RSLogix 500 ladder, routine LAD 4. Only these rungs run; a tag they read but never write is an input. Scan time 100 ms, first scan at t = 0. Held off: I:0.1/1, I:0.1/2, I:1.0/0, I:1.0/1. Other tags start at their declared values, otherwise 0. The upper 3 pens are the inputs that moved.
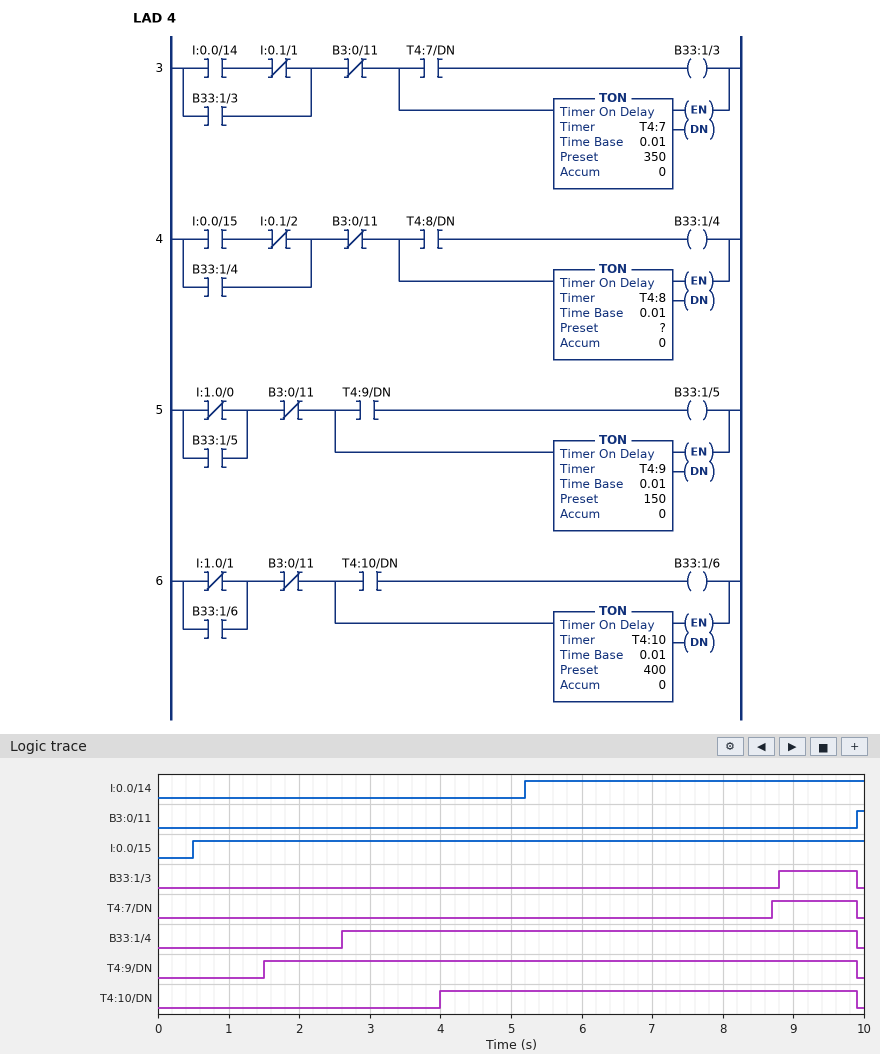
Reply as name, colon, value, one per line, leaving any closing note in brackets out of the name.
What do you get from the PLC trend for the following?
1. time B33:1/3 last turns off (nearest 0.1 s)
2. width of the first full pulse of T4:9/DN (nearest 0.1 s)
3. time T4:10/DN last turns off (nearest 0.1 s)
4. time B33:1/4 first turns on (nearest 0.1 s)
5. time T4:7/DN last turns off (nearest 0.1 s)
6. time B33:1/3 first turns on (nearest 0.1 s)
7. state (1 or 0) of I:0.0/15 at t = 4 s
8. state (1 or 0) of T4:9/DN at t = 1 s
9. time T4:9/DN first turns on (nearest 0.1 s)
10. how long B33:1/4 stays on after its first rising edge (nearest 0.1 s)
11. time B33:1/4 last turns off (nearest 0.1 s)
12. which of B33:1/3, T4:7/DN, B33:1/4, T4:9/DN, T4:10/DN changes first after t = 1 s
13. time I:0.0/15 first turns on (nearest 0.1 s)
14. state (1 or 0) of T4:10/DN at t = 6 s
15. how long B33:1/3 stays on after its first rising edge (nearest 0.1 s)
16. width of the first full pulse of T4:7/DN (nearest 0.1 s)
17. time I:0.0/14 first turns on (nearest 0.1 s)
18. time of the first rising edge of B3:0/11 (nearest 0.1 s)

time B33:1/3 last turns off: 9.9 s
width of the first full pulse of T4:9/DN: 8.4 s
time T4:10/DN last turns off: 9.9 s
time B33:1/4 first turns on: 2.6 s
time T4:7/DN last turns off: 9.9 s
time B33:1/3 first turns on: 8.8 s
state (1 or 0) of I:0.0/15 at t = 4 s: 1
state (1 or 0) of T4:9/DN at t = 1 s: 0
time T4:9/DN first turns on: 1.5 s
how long B33:1/4 stays on after its first rising edge: 7.3 s
time B33:1/4 last turns off: 9.9 s
which of B33:1/3, T4:7/DN, B33:1/4, T4:9/DN, T4:10/DN changes first after t = 1 s: T4:9/DN
time I:0.0/15 first turns on: 0.5 s
state (1 or 0) of T4:10/DN at t = 6 s: 1
how long B33:1/3 stays on after its first rising edge: 1.1 s
width of the first full pulse of T4:7/DN: 1.2 s
time I:0.0/14 first turns on: 5.2 s
time of the first rising edge of B3:0/11: 9.9 s
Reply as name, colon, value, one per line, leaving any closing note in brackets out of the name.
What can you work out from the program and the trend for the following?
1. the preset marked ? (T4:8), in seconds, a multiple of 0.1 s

the preset marked ? (T4:8), in seconds, a multiple of 0.1 s: 2.0 s
